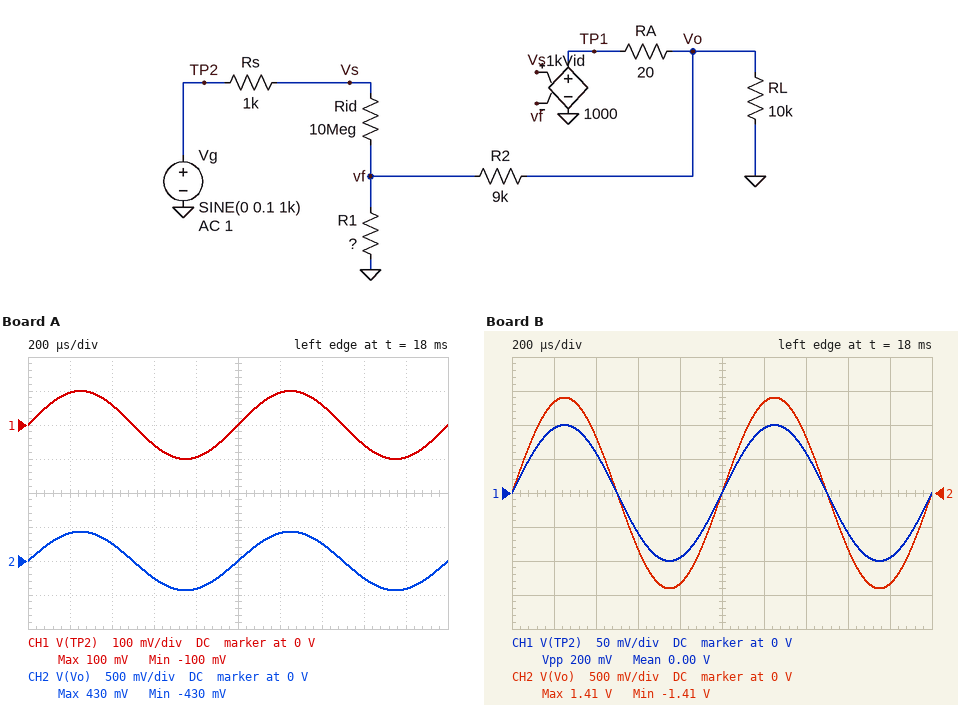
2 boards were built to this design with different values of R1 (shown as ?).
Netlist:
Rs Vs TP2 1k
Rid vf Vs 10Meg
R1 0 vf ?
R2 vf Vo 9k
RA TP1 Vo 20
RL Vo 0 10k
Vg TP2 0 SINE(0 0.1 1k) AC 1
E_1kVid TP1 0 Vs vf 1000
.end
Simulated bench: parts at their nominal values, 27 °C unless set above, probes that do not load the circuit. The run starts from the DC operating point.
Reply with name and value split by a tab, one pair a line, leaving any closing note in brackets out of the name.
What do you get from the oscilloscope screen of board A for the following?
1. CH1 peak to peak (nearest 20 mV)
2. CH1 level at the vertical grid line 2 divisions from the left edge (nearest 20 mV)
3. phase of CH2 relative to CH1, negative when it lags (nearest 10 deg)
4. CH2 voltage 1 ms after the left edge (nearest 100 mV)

CH1 peak to peak	200 mV
CH1 level at the vertical grid line 2 divisions from the left edge	60 mV
phase of CH2 relative to CH1, negative when it lags	0 deg
CH2 voltage 1 ms after the left edge	0 V
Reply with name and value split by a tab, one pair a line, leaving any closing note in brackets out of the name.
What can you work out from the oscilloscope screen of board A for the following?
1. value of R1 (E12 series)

value of R1	2.7 kΩ
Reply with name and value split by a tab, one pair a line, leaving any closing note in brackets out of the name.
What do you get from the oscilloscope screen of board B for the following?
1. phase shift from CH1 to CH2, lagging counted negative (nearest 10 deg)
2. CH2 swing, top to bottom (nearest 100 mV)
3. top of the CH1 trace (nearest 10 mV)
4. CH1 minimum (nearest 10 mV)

phase shift from CH1 to CH2, lagging counted negative	0 deg
CH2 swing, top to bottom	2.8 V
top of the CH1 trace	100 mV
CH1 minimum	-100 mV
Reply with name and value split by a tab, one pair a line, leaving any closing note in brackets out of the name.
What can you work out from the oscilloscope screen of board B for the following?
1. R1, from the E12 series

R1, from the E12 series	680 Ω
